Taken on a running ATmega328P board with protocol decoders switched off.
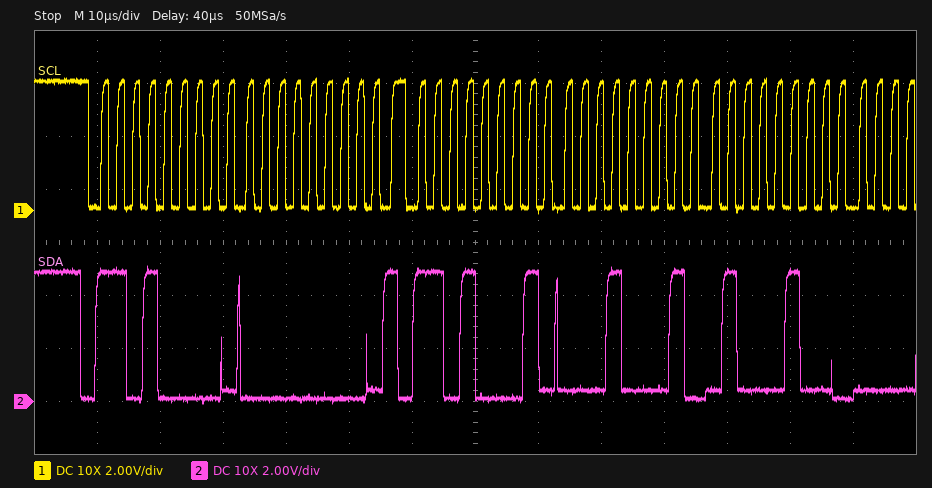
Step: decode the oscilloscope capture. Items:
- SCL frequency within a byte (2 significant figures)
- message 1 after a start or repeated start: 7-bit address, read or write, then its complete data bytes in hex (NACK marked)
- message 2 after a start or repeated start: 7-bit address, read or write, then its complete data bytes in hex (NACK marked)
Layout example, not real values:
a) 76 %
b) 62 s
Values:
a) 400 kHz
b) 0x68 write: 00
c) 0x68 read: 11 44
